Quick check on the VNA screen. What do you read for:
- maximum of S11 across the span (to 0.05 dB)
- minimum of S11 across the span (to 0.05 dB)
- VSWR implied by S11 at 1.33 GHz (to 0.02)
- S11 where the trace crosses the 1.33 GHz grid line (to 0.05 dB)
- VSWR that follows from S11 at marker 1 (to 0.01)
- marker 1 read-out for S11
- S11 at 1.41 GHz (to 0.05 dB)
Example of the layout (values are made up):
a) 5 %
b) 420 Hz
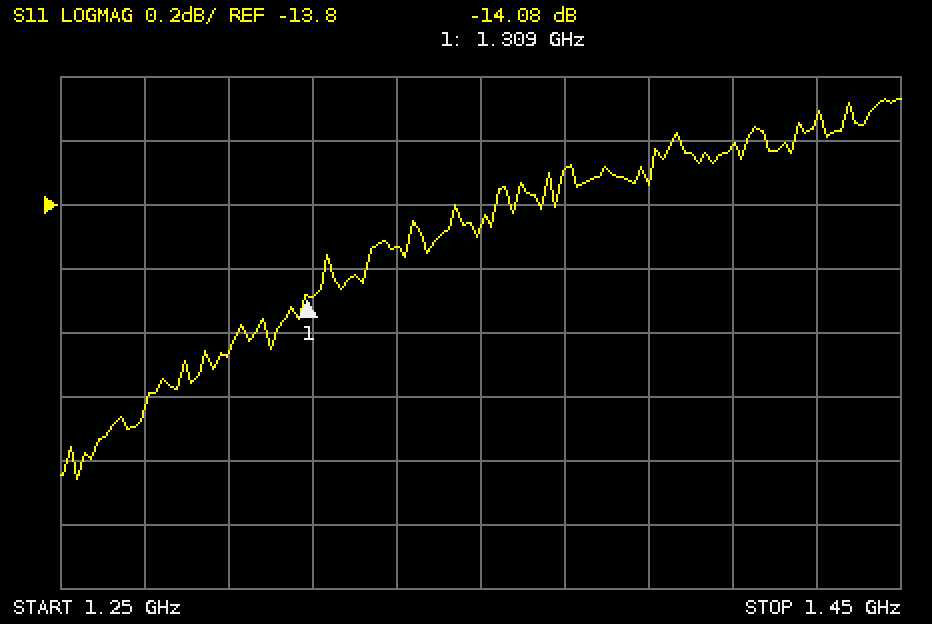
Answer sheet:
a) -13.45 dB
b) -14.65 dB
c) 1.50
d) -13.95 dB
e) 1.49
f) -14.08 dB
g) -13.60 dB
